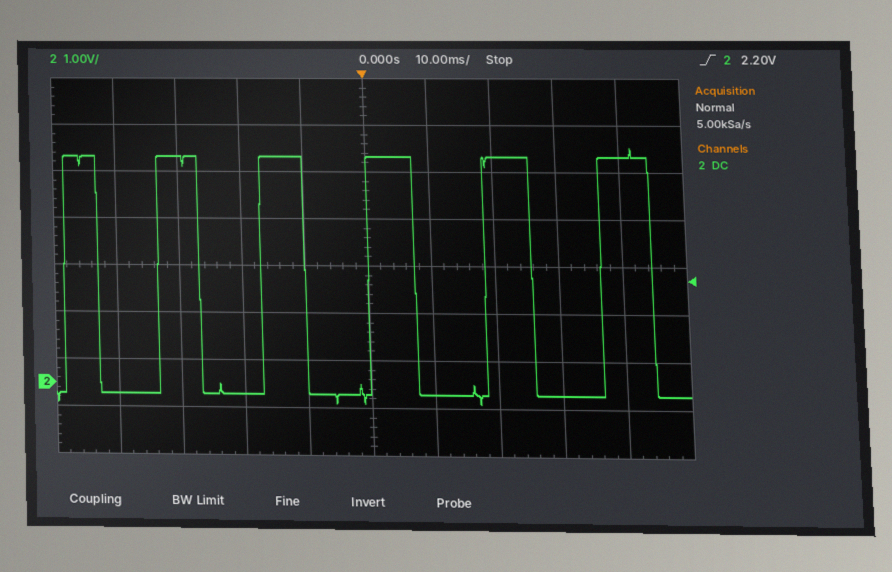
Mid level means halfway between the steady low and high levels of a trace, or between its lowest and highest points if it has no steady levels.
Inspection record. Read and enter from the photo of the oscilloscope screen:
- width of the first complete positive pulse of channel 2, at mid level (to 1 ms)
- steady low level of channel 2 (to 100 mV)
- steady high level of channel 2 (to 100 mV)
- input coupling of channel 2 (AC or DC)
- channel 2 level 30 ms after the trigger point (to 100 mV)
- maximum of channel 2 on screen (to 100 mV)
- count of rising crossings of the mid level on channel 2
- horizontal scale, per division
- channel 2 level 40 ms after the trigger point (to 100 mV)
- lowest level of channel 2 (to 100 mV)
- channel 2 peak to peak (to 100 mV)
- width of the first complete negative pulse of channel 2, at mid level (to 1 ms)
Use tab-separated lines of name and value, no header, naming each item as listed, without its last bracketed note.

width of the first complete positive pulse of channel 2, at mid level	5 ms
steady low level of channel 2	-200 mV
steady high level of channel 2	4.8 V
input coupling of channel 2	DC
channel 2 level 30 ms after the trigger point	-200 mV
maximum of channel 2 on screen	5.0 V
count of rising crossings of the mid level on channel 2	6
horizontal scale, per division	10 ms
channel 2 level 40 ms after the trigger point	4.8 V
lowest level of channel 2	-400 mV
channel 2 peak to peak	5.4 V
width of the first complete negative pulse of channel 2, at mid level	10 ms
